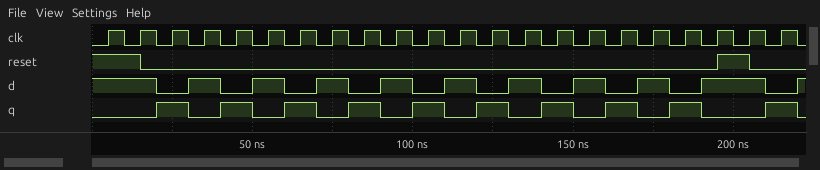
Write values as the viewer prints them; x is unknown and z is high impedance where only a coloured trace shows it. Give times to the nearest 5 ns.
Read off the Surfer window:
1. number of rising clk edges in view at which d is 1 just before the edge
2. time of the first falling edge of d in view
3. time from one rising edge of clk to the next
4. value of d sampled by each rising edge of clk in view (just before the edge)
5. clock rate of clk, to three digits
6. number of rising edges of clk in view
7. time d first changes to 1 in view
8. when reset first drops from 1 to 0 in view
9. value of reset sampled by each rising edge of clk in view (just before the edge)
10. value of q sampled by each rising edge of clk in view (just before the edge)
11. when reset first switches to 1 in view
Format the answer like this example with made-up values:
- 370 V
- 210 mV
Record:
- 12
- 20 ns
- 10 ns
- 1 1 0 1 0 1 0 1 0 1 0 1 0 1 0 1 0 1 0 1 1 0
- 100 MHz
- 22
- 30 ns
- 15 ns
- 1 1 0 0 0 0 0 0 0 0 0 0 0 0 0 0 0 0 0 0 1 0
- 0 0 1 0 1 0 1 0 1 0 1 0 1 0 1 0 1 0 1 0 0 1
- 195 ns
